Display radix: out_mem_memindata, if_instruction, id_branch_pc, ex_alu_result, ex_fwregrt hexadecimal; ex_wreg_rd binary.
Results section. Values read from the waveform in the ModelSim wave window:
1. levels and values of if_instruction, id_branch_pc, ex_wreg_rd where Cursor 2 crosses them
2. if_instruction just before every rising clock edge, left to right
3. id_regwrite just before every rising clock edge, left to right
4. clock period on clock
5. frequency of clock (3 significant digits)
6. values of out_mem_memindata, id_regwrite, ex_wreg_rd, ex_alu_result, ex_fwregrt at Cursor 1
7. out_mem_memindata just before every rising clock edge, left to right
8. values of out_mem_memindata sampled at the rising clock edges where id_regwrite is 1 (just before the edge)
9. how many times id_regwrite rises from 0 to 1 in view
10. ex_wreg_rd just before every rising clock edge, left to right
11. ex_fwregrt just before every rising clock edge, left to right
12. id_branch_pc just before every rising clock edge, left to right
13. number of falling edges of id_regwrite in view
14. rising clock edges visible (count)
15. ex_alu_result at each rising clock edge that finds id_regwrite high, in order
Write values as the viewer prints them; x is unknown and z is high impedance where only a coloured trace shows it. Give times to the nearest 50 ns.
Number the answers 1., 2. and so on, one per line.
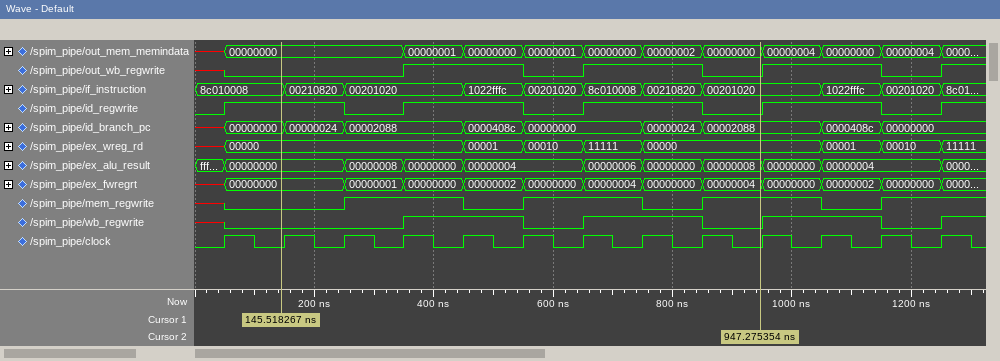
1. if_instruction=00201020, id_branch_pc=00002088, ex_wreg_rd=00000
2. 8c010008, 8c010008, 00210820, 00201020, 00201020, 1022fffc, 00201020, 8c010008, 00210820, 00201020, 00201020, 1022fffc, 00201020
3. 0 1 1 0 1 1 0 1 1 0 1 1 0
4. 100 ns
5. 10.0 MHz
6. out_mem_memindata=00000000, id_regwrite=1, ex_wreg_rd=00000, ex_alu_result=00000000, ex_fwregrt=00000000
7. x, 00000000, 00000000, 00000000, 00000001, 00000000, 00000001, 00000000, 00000002, 00000000, 00000004, 00000000, 00000004
8. 00000000, 00000000, 00000001, 00000000, 00000000, 00000002, 00000004, 00000000
9. 5
10. x, 00000, 00000, 00000, 00000, 00001, 00010, 11111, 00000, 00000, 00000, 00001, 00010
11. x, 00000000, 00000000, 00000001, 00000000, 00000002, 00000000, 00000004, 00000000, 00000004, 00000000, 00000002, 00000000
12. x, 00000000, 00000024, 00002088, 00002088, 0000408c, 00000000, 00000000, 00000024, 00002088, 00002088, 0000408c, 00000000
13. 4
14. 13
15. 00000000, 00000000, 00000000, 00000004, 00000006, 00000000, 00000000, 00000004
